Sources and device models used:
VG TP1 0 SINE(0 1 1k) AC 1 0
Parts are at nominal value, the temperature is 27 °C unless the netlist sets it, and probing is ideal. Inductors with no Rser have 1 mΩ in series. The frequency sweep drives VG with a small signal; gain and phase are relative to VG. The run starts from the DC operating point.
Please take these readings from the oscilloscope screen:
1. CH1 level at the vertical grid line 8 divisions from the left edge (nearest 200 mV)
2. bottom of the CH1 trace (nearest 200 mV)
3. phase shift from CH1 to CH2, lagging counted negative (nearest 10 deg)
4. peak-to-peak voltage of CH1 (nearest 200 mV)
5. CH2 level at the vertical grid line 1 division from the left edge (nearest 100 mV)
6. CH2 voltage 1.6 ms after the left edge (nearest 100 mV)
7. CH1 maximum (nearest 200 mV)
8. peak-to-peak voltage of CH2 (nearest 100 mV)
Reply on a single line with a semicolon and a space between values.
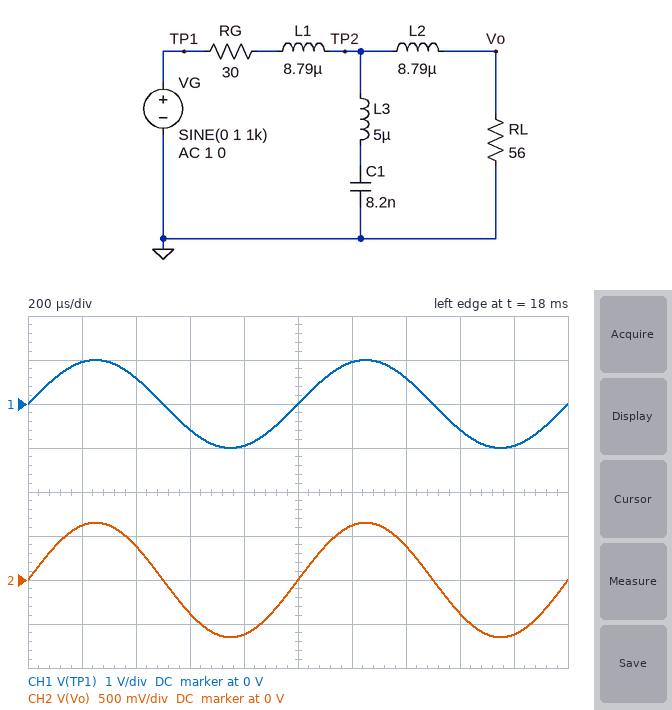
-600 mV; -1.0 V; 0 deg; 2.0 V; 600 mV; -400 mV; 1.0 V; 1.3 V
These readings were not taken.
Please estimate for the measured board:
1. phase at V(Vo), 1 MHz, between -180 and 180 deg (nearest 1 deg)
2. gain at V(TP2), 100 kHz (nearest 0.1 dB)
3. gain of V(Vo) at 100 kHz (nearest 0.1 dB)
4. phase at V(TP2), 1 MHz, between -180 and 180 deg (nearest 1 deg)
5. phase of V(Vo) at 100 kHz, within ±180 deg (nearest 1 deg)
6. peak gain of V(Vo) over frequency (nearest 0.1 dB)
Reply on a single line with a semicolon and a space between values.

-25 deg; -3.7 dB; -3.7 dB; 20 deg; -13 deg; -3.5 dB
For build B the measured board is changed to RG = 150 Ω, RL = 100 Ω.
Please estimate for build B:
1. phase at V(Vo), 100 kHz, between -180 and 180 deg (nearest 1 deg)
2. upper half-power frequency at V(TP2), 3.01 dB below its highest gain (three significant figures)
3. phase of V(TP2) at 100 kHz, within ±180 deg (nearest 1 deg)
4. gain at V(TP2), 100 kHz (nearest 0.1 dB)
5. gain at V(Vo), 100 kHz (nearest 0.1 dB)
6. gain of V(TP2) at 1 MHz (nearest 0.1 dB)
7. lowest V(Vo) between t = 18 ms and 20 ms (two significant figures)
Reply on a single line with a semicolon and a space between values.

-20 deg; 314 kHz; -17 deg; -8.2 dB; -8.3 dB; -23.2 dB; -400 mV
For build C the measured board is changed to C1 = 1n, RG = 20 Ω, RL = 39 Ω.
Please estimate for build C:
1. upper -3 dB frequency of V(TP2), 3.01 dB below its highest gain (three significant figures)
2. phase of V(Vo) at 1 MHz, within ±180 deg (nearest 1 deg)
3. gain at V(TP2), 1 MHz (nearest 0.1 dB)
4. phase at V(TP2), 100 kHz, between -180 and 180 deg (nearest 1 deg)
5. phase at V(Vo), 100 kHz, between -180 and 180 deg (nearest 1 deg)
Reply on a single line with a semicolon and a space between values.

1.71 MHz; -70 deg; -3.3 dB; -3 deg; -11 deg
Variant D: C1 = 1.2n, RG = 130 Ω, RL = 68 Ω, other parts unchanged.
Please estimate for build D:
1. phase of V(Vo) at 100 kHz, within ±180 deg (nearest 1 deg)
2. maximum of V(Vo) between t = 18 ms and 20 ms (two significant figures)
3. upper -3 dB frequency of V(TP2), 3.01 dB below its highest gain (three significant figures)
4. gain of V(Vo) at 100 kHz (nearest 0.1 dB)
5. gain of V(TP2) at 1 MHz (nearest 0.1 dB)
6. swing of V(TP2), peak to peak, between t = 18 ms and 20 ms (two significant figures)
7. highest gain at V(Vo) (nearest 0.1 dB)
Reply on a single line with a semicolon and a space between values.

-5 deg; 340 mV; 1.53 MHz; -9.3 dB; -6.7 dB; 690 mV; -8.9 dB
